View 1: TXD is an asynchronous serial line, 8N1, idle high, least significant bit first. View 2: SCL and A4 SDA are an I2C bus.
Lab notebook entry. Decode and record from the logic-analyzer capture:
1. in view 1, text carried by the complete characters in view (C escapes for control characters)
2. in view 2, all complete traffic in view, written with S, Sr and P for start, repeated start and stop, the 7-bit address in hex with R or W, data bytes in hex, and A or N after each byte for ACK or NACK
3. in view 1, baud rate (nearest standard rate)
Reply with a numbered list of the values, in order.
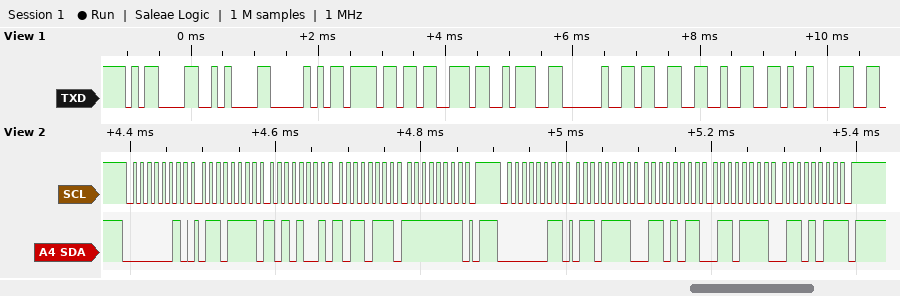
1. "\r\nPos: 32\t"
2. S 01W A 6F A A9 A B7 A FF A P S 01R A 6F A 6B A 6F A 6B N P
3. 9600 baud
